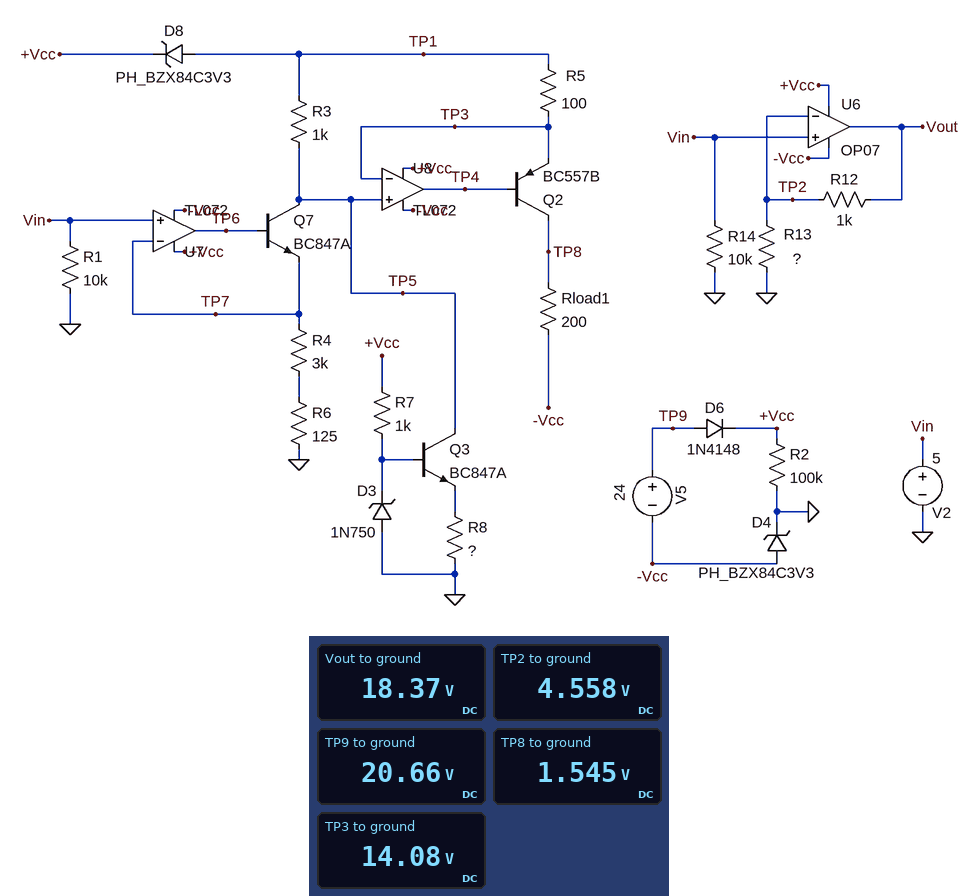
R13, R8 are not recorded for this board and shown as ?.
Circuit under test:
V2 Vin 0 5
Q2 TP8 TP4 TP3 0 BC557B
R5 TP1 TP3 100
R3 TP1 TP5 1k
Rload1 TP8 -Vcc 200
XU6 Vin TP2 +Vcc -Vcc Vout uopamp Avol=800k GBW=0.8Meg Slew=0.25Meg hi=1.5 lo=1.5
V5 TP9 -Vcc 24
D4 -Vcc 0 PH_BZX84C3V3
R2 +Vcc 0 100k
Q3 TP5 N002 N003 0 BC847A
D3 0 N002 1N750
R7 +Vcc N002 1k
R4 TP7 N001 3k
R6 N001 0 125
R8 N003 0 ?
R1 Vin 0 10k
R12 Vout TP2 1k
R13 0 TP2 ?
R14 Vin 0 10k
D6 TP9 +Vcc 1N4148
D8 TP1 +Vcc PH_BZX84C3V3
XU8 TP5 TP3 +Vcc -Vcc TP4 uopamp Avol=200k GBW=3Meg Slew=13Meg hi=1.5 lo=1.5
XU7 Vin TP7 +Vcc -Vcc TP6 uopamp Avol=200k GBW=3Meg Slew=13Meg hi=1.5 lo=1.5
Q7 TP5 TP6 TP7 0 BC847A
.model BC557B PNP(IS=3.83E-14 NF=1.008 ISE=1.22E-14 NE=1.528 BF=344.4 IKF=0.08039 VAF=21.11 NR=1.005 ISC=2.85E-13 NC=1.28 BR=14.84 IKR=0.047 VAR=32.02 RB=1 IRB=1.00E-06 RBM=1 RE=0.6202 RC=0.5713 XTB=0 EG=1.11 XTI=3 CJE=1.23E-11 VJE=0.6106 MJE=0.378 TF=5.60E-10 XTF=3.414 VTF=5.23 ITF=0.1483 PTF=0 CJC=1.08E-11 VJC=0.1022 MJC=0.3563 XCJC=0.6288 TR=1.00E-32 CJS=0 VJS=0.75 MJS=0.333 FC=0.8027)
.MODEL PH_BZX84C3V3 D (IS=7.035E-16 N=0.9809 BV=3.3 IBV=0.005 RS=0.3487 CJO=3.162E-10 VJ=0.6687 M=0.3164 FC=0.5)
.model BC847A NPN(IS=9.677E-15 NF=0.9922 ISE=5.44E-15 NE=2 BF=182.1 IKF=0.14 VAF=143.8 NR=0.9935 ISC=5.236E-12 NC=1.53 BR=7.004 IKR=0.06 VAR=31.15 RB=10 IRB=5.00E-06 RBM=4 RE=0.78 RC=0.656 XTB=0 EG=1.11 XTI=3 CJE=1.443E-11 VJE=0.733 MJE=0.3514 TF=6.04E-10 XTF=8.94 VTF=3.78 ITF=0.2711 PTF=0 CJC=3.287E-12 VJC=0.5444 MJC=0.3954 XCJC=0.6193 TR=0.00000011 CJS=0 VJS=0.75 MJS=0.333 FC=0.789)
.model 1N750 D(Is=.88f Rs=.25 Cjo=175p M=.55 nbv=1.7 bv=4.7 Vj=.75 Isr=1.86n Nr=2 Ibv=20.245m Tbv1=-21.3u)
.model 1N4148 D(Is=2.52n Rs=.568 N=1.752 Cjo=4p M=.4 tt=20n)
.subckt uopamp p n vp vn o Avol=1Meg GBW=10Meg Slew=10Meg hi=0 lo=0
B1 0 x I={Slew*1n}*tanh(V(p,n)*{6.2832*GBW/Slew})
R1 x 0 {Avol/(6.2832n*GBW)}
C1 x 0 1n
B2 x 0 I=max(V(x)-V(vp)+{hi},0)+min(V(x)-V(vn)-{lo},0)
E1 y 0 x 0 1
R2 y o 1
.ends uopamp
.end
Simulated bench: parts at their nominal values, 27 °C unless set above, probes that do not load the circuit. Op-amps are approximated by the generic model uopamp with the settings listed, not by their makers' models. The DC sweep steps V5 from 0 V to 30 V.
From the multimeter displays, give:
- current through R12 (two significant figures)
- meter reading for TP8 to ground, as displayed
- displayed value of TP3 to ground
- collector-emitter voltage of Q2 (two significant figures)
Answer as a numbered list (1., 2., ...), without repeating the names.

1. 14 mA
2. 1.545 V
3. 14.08 V
4. -13 V
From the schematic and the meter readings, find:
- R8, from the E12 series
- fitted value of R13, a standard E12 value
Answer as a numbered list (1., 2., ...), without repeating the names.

1. 4.7 kΩ
2. 330 Ω
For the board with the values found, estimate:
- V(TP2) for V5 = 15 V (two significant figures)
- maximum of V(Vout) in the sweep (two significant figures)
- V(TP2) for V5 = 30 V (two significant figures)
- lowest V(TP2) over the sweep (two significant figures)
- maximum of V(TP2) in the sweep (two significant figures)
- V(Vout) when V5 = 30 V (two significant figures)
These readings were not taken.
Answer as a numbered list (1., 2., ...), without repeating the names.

1. 2.3 V
2. 20 V
3. 5.0 V
4. -210 mV
5. 5.0 V
6. 20 V
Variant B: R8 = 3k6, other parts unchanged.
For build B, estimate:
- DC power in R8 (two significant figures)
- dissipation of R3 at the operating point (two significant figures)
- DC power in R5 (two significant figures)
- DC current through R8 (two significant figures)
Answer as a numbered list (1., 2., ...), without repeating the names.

1. 4.5 mW
2. 7.3 mW
3. 73 mW
4. 1.1 mA
